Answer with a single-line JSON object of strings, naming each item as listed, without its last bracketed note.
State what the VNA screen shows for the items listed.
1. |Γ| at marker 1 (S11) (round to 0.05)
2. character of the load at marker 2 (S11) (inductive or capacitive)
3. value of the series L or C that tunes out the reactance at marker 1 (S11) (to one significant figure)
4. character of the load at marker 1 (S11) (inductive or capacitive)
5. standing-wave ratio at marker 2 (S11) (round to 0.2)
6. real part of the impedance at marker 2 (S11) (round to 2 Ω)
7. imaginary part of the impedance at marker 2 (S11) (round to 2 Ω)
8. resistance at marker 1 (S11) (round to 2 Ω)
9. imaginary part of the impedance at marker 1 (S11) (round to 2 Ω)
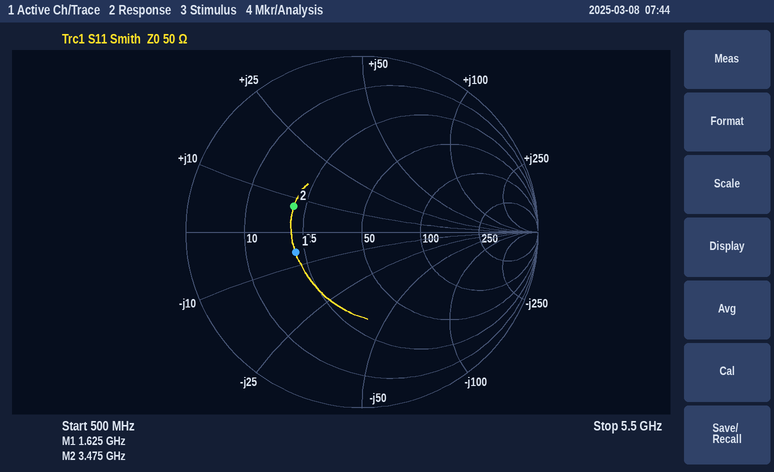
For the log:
{"|Γ| at marker 1 (S11)": "0.40", "character of the load at marker 2 (S11)": "inductive", "value of the series L or C that tunes out the reactance at marker 1 (S11)": "600 pH", "character of the load at marker 1 (S11)": "capacitive", "standing-wave ratio at marker 2 (S11)": "2.4", "real part of the impedance at marker 2 (S11)": "22 Ω", "imaginary part of the impedance at marker 2 (S11)": "+8 Ω", "resistance at marker 1 (S11)": "22 Ω", "imaginary part of the impedance at marker 1 (S11)": "-6 Ω"}
